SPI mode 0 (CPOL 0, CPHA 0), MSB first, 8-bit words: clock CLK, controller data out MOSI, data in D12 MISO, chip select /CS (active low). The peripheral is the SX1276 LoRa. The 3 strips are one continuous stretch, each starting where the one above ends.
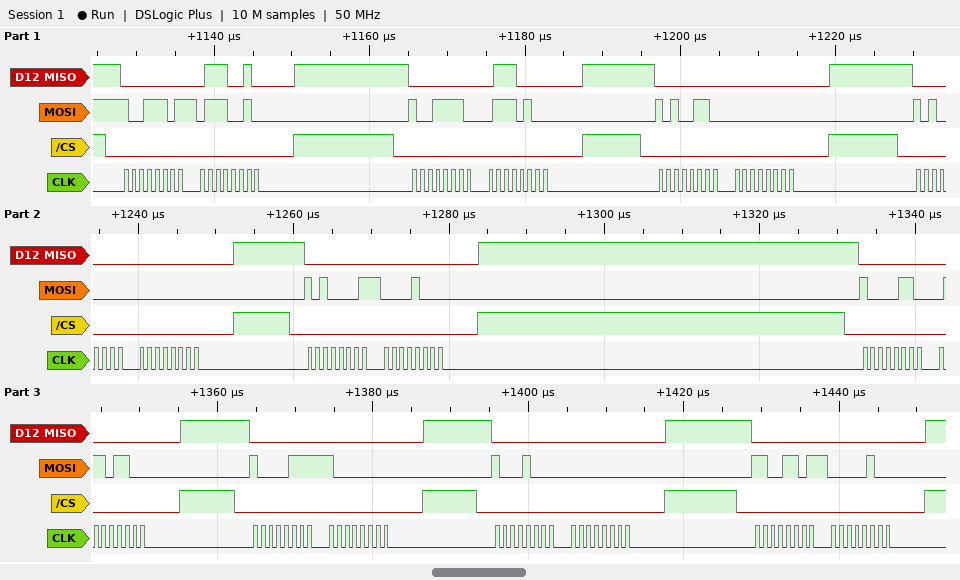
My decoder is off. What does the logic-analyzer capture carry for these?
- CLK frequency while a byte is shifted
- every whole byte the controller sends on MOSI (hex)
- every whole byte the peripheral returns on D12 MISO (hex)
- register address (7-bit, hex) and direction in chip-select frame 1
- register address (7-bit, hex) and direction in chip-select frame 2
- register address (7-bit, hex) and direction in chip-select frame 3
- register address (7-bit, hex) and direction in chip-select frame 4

1 MHz
0x9D 0x72 0x9E 0x74 0xA6 0x00 0xA0 0x00 0xA1 0x08 0x86 0x6C 0x87 0x80 0x88 0x00 0xCD 0x04
0x00 0x72 0x00 0x70 0x00 0x00 0x00 0x00 0x00 0x00 0x00 0x00 0x00 0x00 0x00 0x00 0x00 0x00
0x1D write
0x1E write
0x26 write
0x20 write
